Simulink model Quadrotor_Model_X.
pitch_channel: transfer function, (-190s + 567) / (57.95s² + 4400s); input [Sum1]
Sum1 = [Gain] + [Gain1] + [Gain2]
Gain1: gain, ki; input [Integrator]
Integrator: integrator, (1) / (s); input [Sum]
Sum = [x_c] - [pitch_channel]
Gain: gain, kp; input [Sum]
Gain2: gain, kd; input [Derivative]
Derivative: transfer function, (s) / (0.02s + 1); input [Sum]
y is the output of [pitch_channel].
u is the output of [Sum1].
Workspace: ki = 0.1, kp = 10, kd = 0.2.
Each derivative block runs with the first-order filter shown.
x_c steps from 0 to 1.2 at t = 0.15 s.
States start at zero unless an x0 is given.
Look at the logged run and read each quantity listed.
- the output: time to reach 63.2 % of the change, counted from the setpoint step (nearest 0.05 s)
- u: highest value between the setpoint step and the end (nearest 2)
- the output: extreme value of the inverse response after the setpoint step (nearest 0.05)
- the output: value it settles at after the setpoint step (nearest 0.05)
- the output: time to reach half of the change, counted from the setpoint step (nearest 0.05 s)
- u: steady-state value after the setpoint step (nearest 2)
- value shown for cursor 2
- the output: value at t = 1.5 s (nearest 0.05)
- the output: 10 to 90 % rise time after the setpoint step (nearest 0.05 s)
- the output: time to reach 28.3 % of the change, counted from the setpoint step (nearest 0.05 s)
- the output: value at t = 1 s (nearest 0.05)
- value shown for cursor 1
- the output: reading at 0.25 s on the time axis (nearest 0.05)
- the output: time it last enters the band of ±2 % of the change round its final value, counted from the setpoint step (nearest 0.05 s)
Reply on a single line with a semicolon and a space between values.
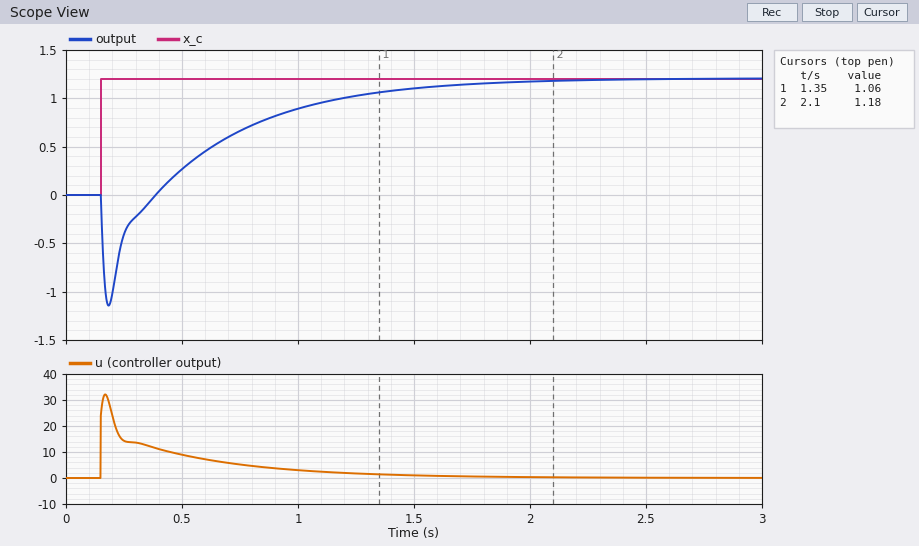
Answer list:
0.70 s; 32; -1.15; 1.20; 0.55 s; 0; 1.18; 1.10; 1.00 s; 0.40 s; 0.90; 1.06; -0.40; 2.00 s
